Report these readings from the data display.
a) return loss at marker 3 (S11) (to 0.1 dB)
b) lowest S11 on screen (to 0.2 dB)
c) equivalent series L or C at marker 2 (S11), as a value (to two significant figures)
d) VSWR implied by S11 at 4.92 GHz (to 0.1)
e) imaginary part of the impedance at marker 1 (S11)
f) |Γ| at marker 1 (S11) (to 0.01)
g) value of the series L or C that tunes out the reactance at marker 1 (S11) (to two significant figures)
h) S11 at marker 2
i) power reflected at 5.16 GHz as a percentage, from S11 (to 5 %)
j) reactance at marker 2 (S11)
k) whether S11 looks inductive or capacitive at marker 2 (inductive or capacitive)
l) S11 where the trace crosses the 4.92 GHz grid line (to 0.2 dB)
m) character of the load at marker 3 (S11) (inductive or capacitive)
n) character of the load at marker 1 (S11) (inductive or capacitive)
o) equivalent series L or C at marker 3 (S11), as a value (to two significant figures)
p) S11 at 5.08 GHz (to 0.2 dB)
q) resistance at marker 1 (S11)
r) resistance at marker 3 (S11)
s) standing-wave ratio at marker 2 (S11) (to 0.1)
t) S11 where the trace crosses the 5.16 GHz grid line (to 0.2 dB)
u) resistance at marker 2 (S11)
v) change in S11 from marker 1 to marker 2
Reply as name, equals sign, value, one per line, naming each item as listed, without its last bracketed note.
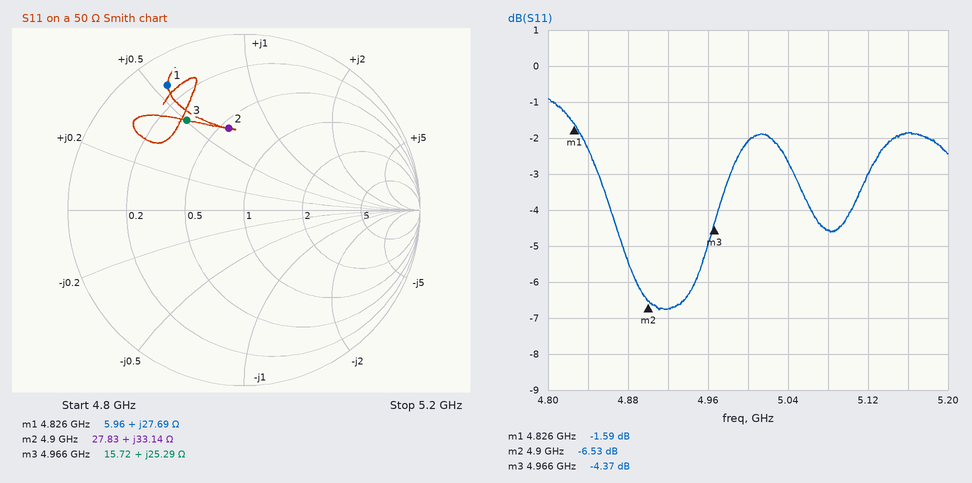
return loss at marker 3 (S11) = 4.4 dB
lowest S11 on screen = -6.8 dB
equivalent series L or C at marker 2 (S11), as a value = 1.1 nH
VSWR implied by S11 at 4.92 GHz = 2.7
imaginary part of the impedance at marker 1 = +27.69 Ω
|Γ| at marker 1 (S11) = 0.83
value of the series L or C that tunes out the reactance at marker 1 (S11) = 1.2 pF
S11 at marker 2 = -6.53 dB
power reflected at 5.16 GHz as a percentage, from S11 = 65 %
reactance at marker 2 = +33.14 Ω
whether S11 looks inductive or capacitive at marker 2 = inductive
S11 where the trace crosses the 4.92 GHz grid line = -6.8 dB
character of the load at marker 3 (S11) = inductive
character of the load at marker 1 (S11) = inductive
equivalent series L or C at marker 3 (S11), as a value = 810 pH
S11 at 5.08 GHz = -4.6 dB
resistance at marker 1 = 5.96 Ω
resistance at marker 3 = 15.72 Ω
standing-wave ratio at marker 2 (S11) = 2.8
S11 where the trace crosses the 5.16 GHz grid line = -1.8 dB
resistance at marker 2 = 27.83 Ω
change in S11 from marker 1 to marker 2 = -4.94 dB
